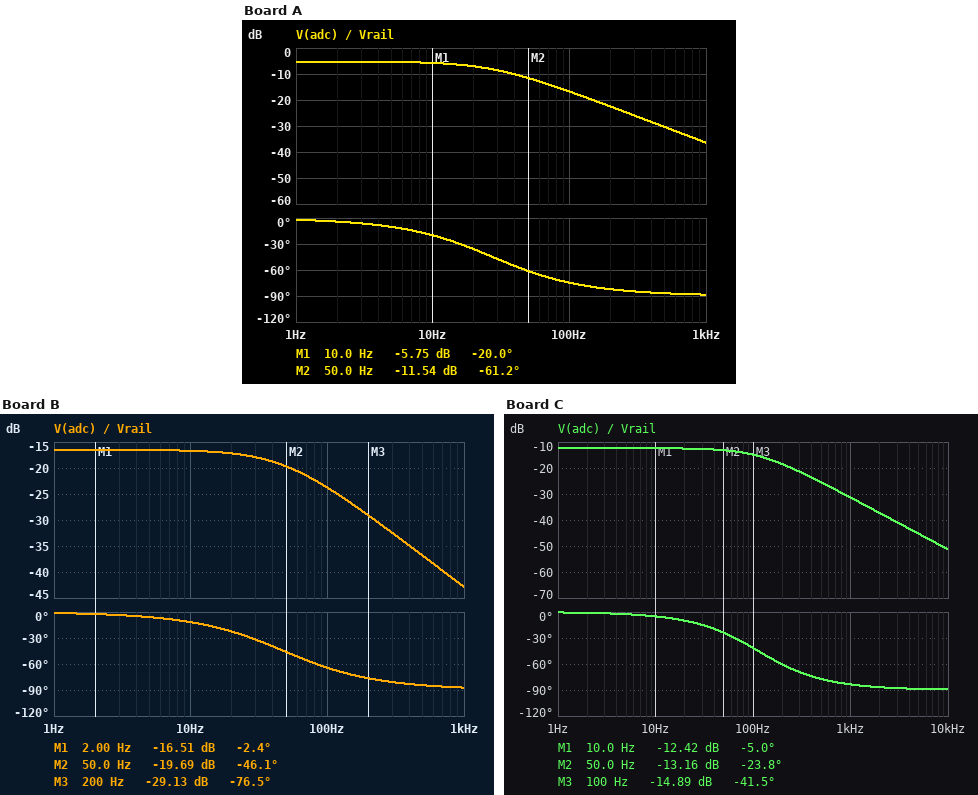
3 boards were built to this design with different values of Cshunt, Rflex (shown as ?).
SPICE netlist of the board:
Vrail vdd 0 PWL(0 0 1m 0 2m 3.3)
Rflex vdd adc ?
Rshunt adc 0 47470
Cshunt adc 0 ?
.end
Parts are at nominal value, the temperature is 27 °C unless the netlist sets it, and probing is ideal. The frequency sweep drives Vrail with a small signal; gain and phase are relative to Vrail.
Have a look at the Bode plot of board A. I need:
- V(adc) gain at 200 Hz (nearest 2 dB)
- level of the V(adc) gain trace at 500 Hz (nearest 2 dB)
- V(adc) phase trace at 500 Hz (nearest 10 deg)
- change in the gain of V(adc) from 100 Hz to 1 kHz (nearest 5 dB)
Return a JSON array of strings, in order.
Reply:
["-22 dB", "-30 dB", "-90 deg", "-20 dB"]
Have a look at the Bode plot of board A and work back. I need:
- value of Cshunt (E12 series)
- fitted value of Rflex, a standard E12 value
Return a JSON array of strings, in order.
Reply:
["270 nF", "39 kΩ"]
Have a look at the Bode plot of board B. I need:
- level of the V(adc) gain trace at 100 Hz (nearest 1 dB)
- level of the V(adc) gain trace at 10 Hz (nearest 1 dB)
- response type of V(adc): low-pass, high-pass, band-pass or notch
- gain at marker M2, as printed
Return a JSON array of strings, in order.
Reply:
["-24 dB", "-17 dB", "low-pass", "-19.69 dB"]
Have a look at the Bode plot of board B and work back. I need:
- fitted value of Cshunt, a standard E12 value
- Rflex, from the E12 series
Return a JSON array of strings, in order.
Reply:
["82 nF", "270 kΩ"]
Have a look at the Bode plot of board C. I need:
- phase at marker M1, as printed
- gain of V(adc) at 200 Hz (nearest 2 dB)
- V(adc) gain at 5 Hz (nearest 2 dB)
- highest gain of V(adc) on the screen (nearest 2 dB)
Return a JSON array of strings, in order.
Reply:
["-5.0 deg", "-18 dB", "-12 dB", "-12 dB"]
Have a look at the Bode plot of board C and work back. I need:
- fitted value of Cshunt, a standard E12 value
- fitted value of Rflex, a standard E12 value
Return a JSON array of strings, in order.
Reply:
["39 nF", "150 kΩ"]
